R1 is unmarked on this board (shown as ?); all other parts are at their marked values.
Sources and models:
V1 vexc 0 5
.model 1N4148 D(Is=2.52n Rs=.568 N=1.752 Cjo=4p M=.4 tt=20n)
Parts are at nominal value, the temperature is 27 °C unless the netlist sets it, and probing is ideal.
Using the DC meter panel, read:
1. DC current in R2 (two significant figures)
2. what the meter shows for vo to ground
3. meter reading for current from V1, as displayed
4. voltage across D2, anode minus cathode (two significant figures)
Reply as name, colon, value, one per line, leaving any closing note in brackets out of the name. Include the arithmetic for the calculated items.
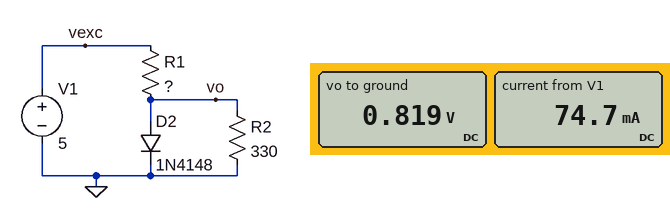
DC current in R2: (819 mV) / 330 Ω = 2.5 mA
what the meter shows for vo to ground: 0.819 V
meter reading for current from V1, as displayed: 74.7 mA
voltage across D2, anode minus cathode: 819 mV = 820 mV
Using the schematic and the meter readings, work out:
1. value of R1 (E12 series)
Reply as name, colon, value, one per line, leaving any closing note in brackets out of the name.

value of R1: 56 Ω
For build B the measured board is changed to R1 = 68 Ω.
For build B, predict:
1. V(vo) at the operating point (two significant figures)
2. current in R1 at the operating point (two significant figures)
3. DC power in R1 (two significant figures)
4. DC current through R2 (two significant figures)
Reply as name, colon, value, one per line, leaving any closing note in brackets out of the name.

V(vo) at the operating point: 800 mV
current in R1 at the operating point: 62 mA
DC power in R1: 260 mW
DC current through R2: 2.4 mA
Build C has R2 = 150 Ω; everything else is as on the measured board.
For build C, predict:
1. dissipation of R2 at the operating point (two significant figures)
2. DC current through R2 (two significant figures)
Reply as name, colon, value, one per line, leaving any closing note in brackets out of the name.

dissipation of R2 at the operating point: 4.4 mW
DC current through R2: 5.4 mA
